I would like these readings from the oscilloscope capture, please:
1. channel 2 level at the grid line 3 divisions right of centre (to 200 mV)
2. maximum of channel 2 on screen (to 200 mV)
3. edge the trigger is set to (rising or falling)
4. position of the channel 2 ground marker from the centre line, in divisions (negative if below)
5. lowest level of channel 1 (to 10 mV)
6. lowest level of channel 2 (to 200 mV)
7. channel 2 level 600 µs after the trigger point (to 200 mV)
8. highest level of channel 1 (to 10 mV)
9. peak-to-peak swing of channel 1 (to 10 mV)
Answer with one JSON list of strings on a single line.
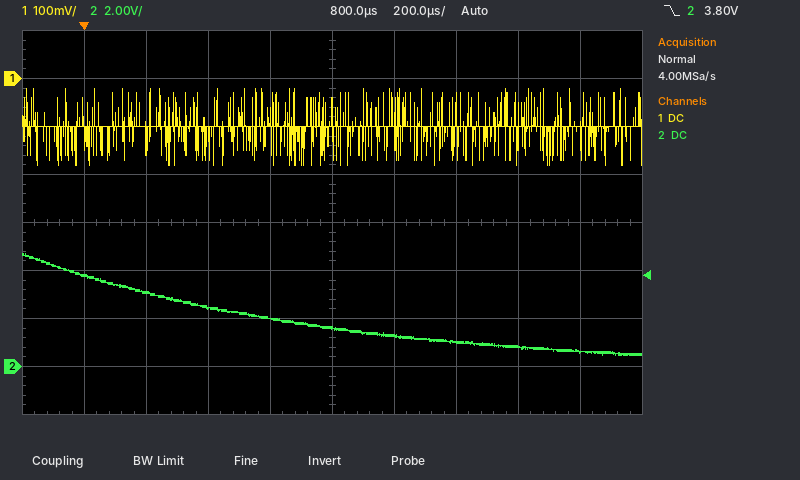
["800 mV", "4.8 V", "falling", "-3.0 div", "-180 mV", "400 mV", "2.0 V", "-20 mV", "160 mV"]
